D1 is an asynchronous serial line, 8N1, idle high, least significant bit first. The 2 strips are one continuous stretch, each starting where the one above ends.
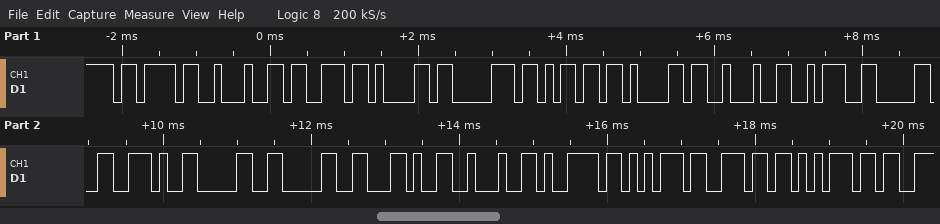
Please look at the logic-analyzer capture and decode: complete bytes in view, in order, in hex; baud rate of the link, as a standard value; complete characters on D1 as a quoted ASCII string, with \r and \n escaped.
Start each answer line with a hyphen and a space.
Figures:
- 7B 22 73 61 70 6D 61 22 3A 30 2E 30 30 2C 22 79 75 6E 75
- 9600 baud
- "{\"sapma\":0.00,\"yunu"
